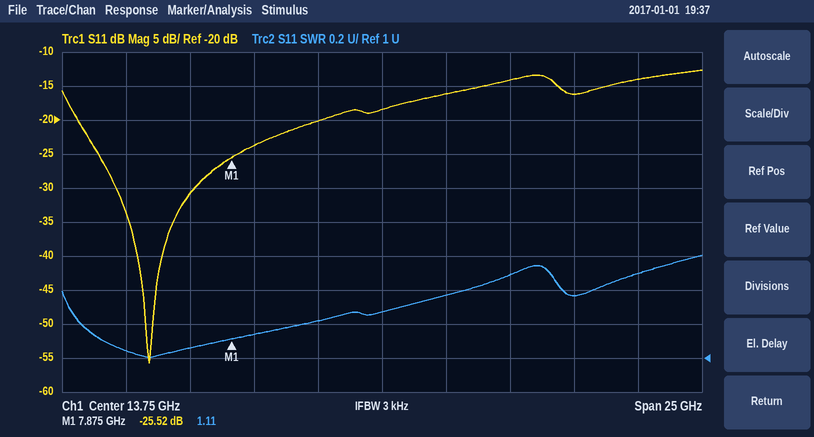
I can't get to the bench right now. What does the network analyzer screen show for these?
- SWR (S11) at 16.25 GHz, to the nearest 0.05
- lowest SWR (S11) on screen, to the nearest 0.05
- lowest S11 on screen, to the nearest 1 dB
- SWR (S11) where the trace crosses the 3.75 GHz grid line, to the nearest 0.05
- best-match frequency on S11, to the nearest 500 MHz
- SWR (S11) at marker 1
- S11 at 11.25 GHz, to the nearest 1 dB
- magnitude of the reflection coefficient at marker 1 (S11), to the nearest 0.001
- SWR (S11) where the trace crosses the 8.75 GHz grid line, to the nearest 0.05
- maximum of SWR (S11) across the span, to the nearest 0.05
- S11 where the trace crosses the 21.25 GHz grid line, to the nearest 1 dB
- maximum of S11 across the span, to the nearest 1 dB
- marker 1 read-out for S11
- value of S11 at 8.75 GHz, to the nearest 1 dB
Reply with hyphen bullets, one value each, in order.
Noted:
- 1.35
- 1.00
- -56 dB
- 1.05
- 4.5 GHz
- 1.11
- -20 dB
- 0.053
- 1.15
- 1.60
- -16 dB
- -13 dB
- -25.52 dB
- -24 dB
